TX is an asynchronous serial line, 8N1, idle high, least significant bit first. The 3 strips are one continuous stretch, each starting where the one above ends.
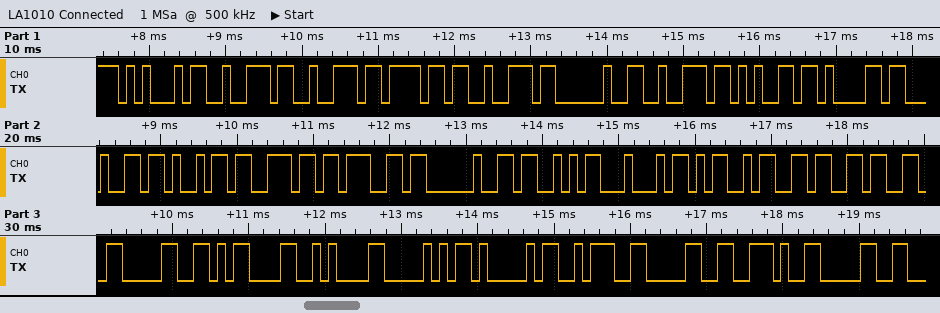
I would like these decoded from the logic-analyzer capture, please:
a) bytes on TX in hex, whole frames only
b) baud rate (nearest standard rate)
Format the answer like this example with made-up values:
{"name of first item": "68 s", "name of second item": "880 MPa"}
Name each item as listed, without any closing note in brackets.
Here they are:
{"bytes on TX in hex, whole frames only": "0x45 0x72 0x72 0x6F 0x72 0x20 0x72 0x65 0x61 0x64 0x69 0x6E 0x67 0x20 0x53 0x44 0x4D 0x36 0x33 0x30 0x0D 0x0A 0x50 0x41 0x3A 0x30 0x2E 0x30", "baud rate": "9600 baud"}
